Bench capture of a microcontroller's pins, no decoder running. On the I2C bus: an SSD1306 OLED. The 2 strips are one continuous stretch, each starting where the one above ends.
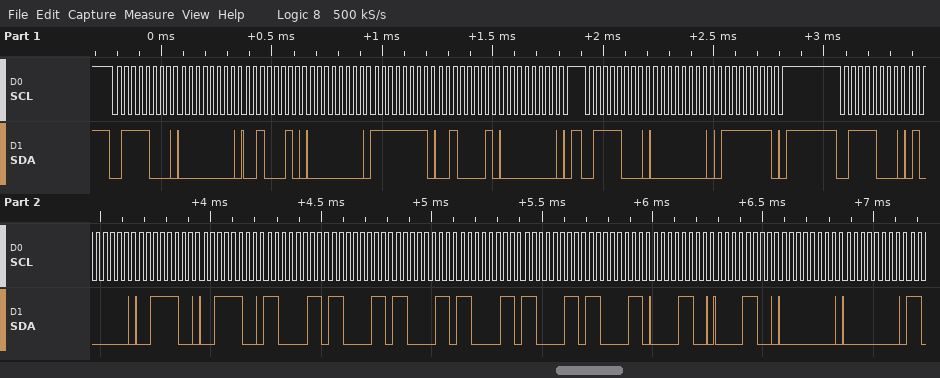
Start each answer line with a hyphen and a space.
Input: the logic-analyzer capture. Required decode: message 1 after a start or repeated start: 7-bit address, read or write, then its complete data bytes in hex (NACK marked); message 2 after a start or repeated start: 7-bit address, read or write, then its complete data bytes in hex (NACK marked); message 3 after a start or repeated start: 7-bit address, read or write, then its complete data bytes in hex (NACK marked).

- 0x3C write: 00 22 00 FF 21 00
- 0x3C write: 00 7F
- 0x3C write: 40 3C 3C C3 C3 C3 C3 C3 C3 0C 0C 00 00
